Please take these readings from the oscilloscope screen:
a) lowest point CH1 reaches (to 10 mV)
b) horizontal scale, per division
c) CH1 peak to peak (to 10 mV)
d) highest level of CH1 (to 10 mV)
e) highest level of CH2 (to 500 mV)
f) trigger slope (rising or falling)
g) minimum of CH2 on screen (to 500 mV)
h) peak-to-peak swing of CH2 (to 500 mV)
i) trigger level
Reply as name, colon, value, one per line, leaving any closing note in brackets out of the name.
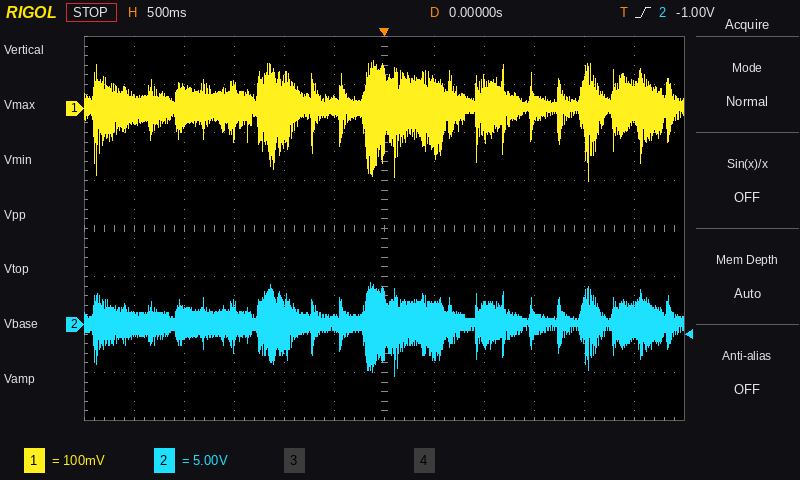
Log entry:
lowest point CH1 reaches: -150 mV
horizontal scale, per division: 500 ms
CH1 peak to peak: 250 mV
highest level of CH1: 100 mV
highest level of CH2: 4.5 V
trigger slope: rising
minimum of CH2 on screen: -5.5 V
peak-to-peak swing of CH2: 10.0 V
trigger level: -1.00 V
